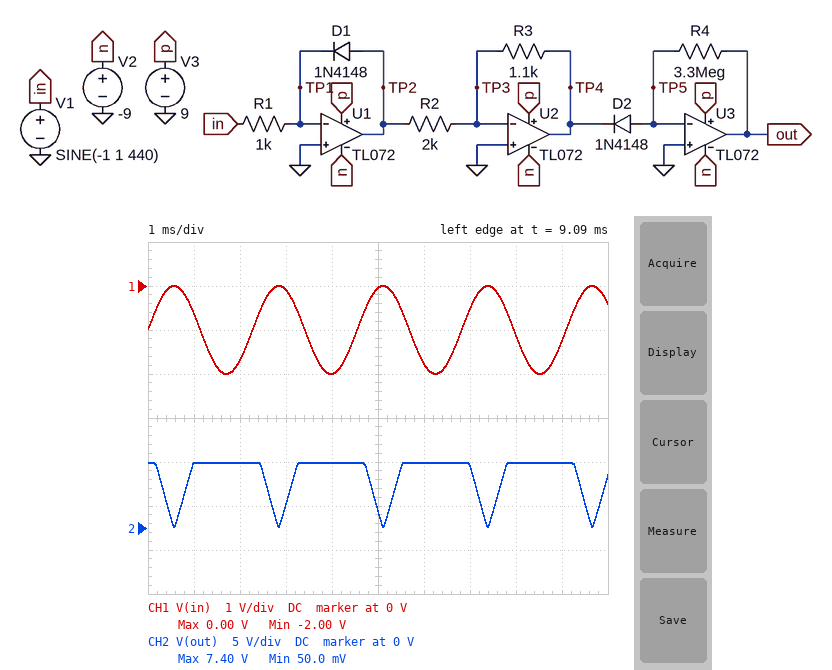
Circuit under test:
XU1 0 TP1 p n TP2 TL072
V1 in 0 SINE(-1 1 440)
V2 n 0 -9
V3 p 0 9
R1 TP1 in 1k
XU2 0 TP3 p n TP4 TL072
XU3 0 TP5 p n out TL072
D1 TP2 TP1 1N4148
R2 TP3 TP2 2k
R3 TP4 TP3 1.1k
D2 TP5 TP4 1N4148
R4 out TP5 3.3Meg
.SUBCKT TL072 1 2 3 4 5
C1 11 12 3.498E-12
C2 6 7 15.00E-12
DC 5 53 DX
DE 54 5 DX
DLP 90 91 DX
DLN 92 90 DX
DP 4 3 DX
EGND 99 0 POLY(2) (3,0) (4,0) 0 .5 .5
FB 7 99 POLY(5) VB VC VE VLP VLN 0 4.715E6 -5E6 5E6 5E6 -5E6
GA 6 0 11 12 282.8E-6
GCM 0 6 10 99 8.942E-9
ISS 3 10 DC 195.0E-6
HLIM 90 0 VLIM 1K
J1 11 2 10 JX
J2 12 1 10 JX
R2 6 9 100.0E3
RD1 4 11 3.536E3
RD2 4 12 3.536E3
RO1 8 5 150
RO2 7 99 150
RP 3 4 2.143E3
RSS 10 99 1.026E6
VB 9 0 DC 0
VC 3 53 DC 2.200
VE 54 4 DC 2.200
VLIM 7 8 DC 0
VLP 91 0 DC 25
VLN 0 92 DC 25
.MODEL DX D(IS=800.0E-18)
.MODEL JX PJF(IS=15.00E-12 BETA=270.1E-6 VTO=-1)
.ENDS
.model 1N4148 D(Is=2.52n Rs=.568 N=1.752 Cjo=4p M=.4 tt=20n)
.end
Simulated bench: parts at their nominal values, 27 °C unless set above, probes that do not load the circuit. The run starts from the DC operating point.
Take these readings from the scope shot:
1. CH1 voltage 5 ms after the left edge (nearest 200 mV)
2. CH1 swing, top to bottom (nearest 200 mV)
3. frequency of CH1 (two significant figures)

0 V
2.0 V
440 Hz
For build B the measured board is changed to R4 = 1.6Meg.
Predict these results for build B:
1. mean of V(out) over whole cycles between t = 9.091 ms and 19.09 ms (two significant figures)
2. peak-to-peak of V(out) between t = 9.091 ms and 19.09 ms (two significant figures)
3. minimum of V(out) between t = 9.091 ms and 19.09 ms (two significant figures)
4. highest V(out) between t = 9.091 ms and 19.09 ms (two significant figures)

4.4 V
7.1 V
29 mV
7.2 V
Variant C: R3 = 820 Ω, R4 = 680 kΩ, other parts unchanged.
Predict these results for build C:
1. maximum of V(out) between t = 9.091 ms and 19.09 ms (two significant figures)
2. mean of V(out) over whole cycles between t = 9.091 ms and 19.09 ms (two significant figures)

450 mV
300 mV
